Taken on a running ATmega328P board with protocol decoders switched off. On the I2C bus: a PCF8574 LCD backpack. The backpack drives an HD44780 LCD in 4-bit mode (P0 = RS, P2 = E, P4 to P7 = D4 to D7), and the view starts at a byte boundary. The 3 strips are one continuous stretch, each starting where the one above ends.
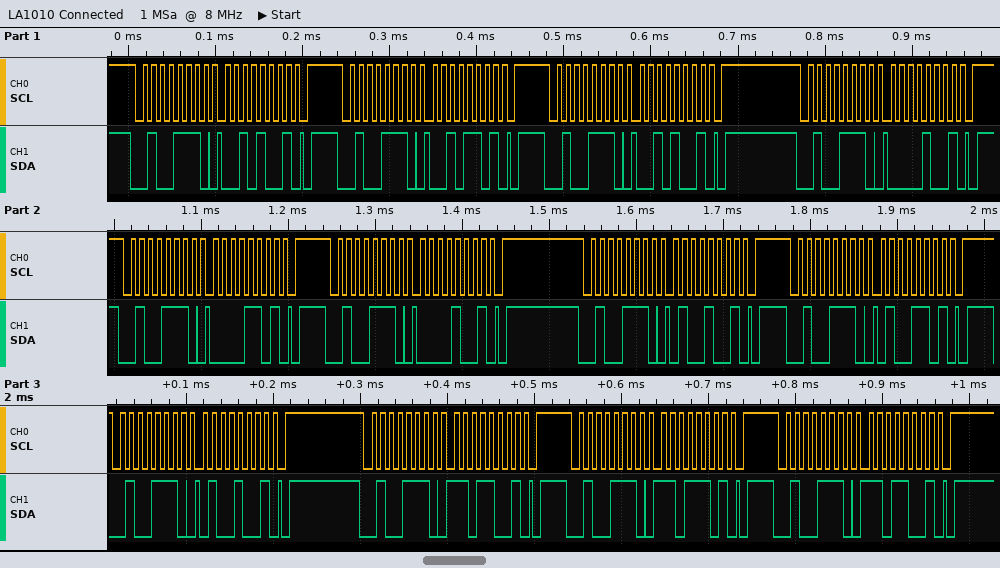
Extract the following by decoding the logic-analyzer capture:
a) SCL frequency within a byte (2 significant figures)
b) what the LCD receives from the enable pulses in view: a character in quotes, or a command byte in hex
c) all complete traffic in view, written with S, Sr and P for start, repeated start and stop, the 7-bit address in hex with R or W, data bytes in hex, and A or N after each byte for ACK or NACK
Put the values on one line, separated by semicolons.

100 kHz; ' ' 'M'; S 27W A 29 A P S 27W A 2D A P S 27W A 29 A P S 27W A 09 A P S 27W A 0D A P S 27W A 09 A P S 27W A 49 A P S 27W A 4D A P S 27W A 49 A P S 27W A D9 A P S 27W A DD A P S 27W A D9 A P
